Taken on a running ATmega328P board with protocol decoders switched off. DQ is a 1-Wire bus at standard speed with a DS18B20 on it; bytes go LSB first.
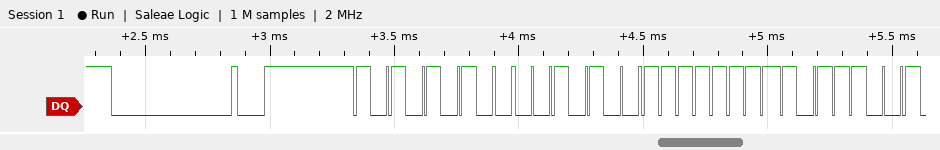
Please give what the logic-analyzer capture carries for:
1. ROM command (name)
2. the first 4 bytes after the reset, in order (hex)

Match ROM
55 28 FF 9D
